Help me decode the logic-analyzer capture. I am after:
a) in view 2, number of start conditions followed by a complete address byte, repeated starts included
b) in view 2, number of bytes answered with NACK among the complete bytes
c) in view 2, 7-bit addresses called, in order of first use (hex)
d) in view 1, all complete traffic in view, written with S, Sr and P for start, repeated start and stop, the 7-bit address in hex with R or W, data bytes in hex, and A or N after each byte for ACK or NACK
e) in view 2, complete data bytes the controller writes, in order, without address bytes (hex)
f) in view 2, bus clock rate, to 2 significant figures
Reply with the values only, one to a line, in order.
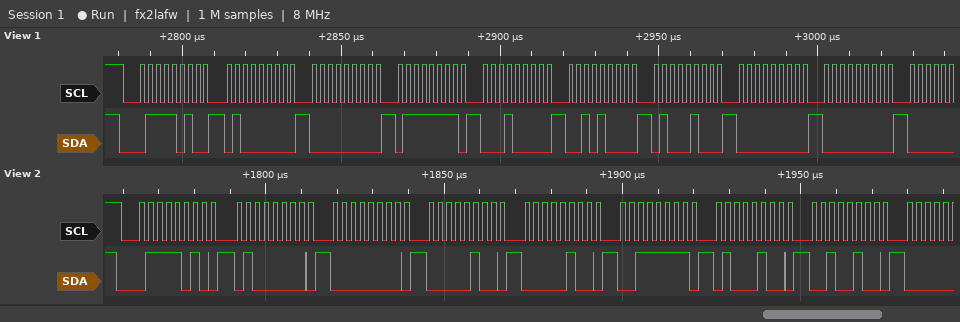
1
0
0x3D
S 3DW A 40 A 00 A 7F A 10 A 28 A 44 A 00 A 00 A
40 00 04 04 3F 44 24
400 kHz
